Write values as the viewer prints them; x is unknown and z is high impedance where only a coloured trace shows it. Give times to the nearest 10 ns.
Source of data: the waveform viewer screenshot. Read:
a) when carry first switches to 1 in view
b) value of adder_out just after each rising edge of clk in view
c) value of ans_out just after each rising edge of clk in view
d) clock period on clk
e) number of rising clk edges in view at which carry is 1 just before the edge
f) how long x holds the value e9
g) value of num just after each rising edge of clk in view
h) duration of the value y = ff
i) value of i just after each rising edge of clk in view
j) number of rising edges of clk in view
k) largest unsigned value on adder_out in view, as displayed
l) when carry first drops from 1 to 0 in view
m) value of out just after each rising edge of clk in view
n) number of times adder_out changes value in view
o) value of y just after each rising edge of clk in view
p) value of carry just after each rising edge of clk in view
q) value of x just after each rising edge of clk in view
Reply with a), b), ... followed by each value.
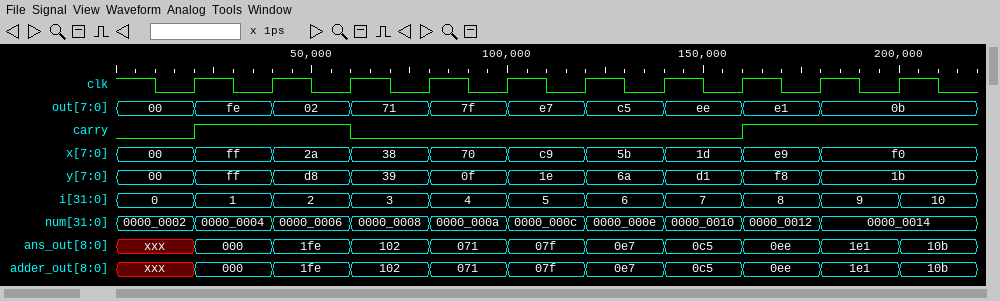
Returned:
a) 20 ns
b) 000, 1fe, 102, 071, 07f, 0e7, 0c5, 0ee, 1e1, 10b
c) 000, 1fe, 102, 071, 07f, 0e7, 0c5, 0ee, 1e1, 10b
d) 20 ns
e) 4
f) 20 ns
g) 0000_0004, 0000_0006, 0000_0008, 0000_000a, 0000_000c, 0000_000e, 0000_0010, 0000_0012, 0000_0014, 0000_0014
h) 20 ns
i) 1, 2, 3, 4, 5, 6, 7, 8, 9, 10
j) 10
k) 1fe
l) 60 ns
m) fe, 02, 71, 7f, e7, c5, ee, e1, 0b, 0b
n) 10
o) ff, d8, 39, 0f, 1e, 6a, d1, f8, 1b, 1b
p) 1 1 0 0 0 0 0 1 1 1
q) ff, 2a, 38, 70, c9, 5b, 1d, e9, f0, f0
